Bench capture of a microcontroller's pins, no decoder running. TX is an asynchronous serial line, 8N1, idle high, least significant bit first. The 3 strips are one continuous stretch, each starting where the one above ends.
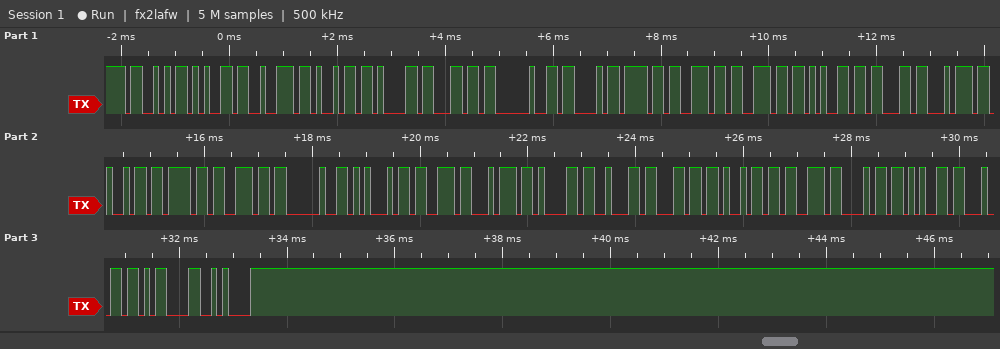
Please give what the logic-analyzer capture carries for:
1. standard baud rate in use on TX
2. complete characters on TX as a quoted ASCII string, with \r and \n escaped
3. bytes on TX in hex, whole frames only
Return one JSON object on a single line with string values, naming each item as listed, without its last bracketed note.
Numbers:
{"standard baud rate in use on TX": "9600 baud", "complete characters on TX as a quoted ASCII string, with \\r and \\n escaped": "\"Serial Connection Established\\r\\n\"", "bytes on TX in hex, whole frames only": "53 65 72 69 61 6C 20 43 6F 6E 6E 65 63 74 69 6F 6E 20 45 73 74 61 62 6C 69 73 68 65 64 0D 0A"}
